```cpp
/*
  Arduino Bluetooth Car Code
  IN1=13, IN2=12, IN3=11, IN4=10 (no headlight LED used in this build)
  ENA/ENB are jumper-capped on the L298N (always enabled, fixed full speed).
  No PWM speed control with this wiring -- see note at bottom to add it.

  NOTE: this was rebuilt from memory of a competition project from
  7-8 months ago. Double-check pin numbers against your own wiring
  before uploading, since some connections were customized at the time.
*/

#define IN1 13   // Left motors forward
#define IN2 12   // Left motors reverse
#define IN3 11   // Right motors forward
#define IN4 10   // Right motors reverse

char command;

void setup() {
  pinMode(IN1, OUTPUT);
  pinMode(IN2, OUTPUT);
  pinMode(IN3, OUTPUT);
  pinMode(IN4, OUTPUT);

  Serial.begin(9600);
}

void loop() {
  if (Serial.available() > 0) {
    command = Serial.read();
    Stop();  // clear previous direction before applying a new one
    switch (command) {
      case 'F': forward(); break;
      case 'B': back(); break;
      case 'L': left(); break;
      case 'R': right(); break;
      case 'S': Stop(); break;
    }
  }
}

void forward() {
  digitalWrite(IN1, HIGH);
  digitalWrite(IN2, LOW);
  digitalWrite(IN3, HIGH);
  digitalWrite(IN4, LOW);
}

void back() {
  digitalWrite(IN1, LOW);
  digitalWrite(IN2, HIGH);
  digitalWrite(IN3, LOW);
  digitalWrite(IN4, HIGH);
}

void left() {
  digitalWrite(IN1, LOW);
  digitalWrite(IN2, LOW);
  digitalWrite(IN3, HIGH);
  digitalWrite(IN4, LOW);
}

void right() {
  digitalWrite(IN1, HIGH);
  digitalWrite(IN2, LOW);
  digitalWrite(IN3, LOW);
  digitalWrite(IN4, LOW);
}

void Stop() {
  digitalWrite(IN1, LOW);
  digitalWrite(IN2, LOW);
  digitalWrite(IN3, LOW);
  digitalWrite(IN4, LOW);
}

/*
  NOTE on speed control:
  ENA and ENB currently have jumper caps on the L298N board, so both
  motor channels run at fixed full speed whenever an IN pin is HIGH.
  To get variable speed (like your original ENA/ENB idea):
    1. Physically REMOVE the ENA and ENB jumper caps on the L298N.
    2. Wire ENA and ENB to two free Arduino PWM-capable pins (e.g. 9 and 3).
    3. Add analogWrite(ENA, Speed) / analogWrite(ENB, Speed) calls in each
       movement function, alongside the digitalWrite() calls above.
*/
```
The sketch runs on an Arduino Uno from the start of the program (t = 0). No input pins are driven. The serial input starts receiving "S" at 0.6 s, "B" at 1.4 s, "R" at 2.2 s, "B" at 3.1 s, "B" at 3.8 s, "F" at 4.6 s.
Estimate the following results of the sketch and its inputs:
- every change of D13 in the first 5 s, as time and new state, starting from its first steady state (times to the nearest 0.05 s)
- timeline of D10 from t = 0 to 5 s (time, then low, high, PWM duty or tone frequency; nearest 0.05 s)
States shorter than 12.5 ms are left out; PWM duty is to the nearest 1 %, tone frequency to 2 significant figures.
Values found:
0 s low; 2.2 s high; 3.1 s low; 4.6 s high
0 s low; 1.4 s high; 2.2 s low; 3.1 s high; 4.6 s low
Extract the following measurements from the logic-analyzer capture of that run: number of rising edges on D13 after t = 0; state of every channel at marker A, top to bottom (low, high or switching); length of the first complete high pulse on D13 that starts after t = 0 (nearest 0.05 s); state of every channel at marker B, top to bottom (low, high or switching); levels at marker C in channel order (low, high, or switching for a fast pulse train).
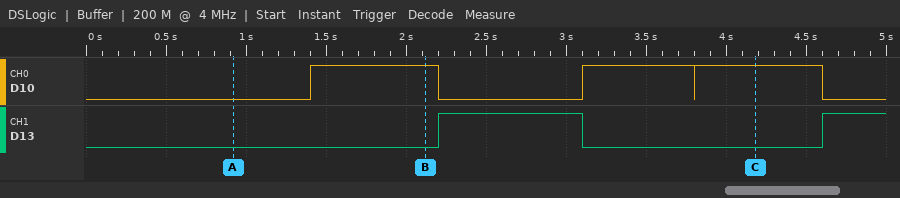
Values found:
2
D10 low, D13 low
0.90 s
D10 high, D13 low
D10 high, D13 low
